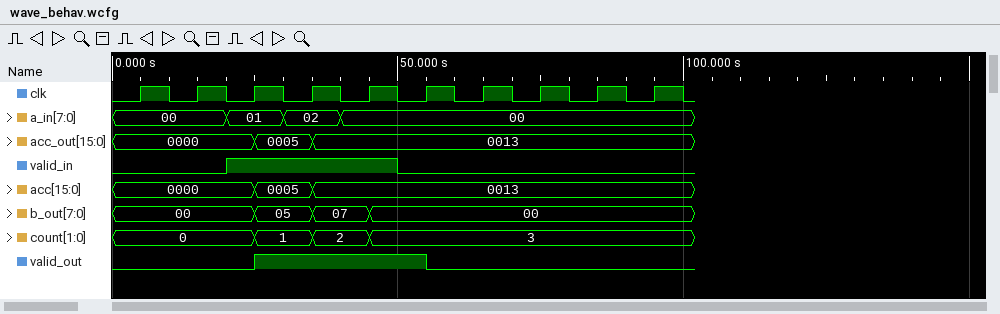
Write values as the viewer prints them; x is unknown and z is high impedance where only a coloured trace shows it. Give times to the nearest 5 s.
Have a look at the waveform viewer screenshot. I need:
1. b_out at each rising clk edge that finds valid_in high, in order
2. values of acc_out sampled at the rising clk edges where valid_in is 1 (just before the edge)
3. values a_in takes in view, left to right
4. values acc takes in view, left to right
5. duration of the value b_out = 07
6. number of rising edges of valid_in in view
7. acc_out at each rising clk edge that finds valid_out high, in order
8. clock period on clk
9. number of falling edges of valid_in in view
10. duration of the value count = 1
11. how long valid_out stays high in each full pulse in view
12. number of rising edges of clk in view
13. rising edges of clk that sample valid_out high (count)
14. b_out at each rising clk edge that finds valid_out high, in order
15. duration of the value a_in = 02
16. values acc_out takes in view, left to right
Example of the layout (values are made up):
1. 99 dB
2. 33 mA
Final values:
1. 00, 05, 07
2. 0000, 0005, 0013
3. 00, 01, 02, 00
4. 0000, 0005, 0013
5. 10 s
6. 1
7. 0005, 0013, 0013
8. 10 s
9. 1
10. 10 s
11. 30 s
12. 10
13. 3
14. 05, 07, 00
15. 10 s
16. 0000, 0005, 0013
